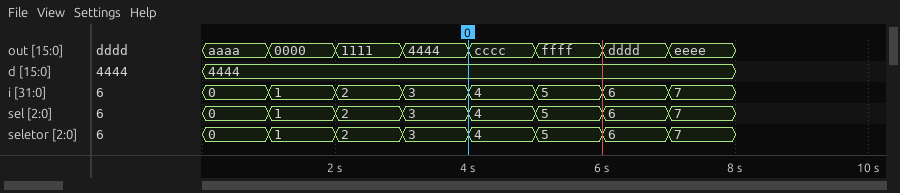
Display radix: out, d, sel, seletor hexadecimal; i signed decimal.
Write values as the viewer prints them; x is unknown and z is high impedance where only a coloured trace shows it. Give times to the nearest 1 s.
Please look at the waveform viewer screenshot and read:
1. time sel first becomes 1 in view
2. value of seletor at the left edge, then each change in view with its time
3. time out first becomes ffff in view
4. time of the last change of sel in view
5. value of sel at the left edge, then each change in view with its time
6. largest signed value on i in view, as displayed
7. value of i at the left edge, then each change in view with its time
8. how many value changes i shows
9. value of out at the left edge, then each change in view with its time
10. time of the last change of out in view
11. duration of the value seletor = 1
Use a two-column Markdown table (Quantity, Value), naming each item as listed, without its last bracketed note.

| Quantity | Value |
|---|---|
| time sel first becomes 1 in view | 1 s |
| value of seletor at the left edge, then each change in view with its time | 0, 1 at 1 s, 2 at 2 s, 3 at 3 s, 4 at 4 s, 5 at 5 s, 6 at 6 s, 7 at 7 s |
| time out first becomes ffff in view | 5 s |
| time of the last change of sel in view | 7 s |
| value of sel at the left edge, then each change in view with its time | 0, 1 at 1 s, 2 at 2 s, 3 at 3 s, 4 at 4 s, 5 at 5 s, 6 at 6 s, 7 at 7 s |
| largest signed value on i in view, as displayed | 7 |
| value of i at the left edge, then each change in view with its time | 0, 1 at 1 s, 2 at 2 s, 3 at 3 s, 4 at 4 s, 5 at 5 s, 6 at 6 s, 7 at 7 s |
| how many value changes i shows | 7 |
| value of out at the left edge, then each change in view with its time | aaaa, 0000 at 1 s, 1111 at 2 s, 4444 at 3 s, cccc at 4 s, ffff at 5 s, dddd at 6 s, eeee at 7 s |
| time of the last change of out in view | 7 s |
| duration of the value seletor = 1 | 1 s |
